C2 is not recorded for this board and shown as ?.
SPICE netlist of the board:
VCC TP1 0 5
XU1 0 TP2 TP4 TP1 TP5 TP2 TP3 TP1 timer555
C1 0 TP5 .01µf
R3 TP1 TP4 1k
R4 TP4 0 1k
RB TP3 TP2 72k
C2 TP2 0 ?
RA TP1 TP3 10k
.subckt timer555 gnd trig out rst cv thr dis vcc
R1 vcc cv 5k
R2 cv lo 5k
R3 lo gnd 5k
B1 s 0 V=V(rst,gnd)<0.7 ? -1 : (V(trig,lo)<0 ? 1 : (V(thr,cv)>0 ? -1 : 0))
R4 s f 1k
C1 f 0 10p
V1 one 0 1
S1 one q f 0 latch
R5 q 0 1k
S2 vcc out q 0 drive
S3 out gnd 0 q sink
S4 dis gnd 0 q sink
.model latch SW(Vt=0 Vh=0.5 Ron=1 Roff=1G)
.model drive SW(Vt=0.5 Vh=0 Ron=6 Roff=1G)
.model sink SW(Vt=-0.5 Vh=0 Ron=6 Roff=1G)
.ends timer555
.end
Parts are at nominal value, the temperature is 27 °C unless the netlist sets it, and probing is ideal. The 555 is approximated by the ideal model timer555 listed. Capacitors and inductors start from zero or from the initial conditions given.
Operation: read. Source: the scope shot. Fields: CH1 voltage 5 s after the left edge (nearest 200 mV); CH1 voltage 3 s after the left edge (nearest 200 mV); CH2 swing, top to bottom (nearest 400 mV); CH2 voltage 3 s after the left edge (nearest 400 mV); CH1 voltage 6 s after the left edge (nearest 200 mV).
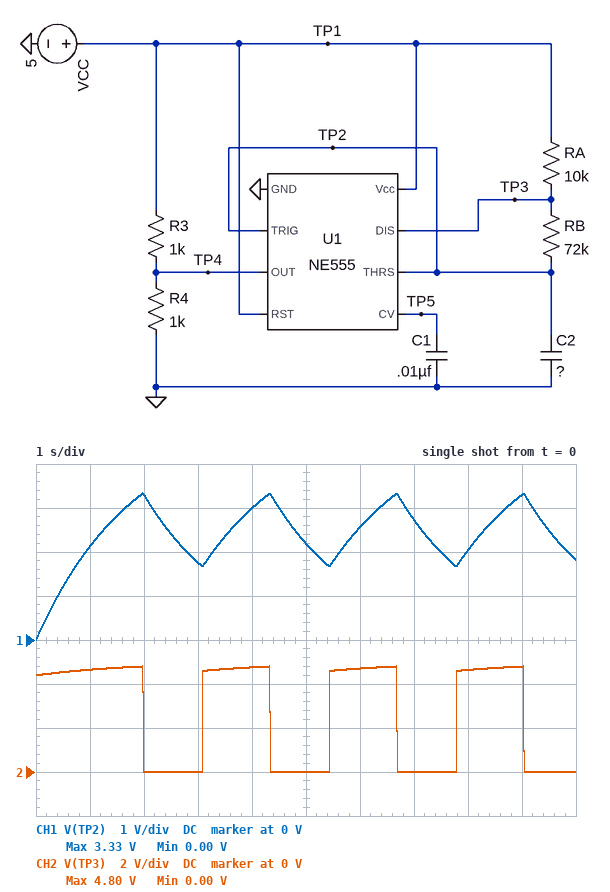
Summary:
2.2 V
1.8 V
4.8 V
0 V
2.6 V
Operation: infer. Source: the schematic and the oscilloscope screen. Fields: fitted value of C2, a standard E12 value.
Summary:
22 µF
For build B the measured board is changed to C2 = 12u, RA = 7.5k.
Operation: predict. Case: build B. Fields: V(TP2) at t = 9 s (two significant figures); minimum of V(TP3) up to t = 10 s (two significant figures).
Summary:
2.1 V
4.1 mV
